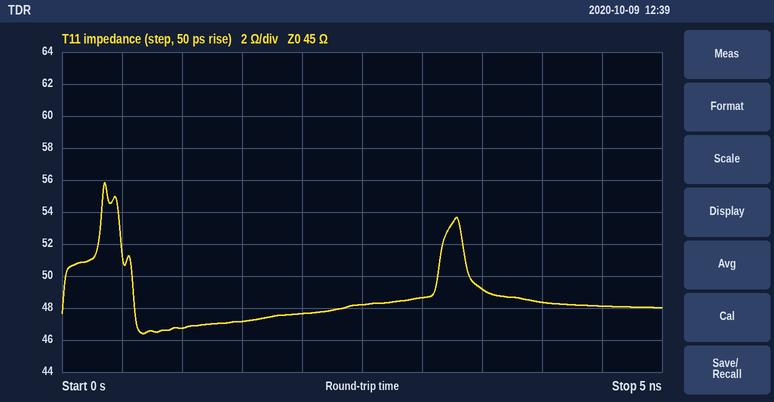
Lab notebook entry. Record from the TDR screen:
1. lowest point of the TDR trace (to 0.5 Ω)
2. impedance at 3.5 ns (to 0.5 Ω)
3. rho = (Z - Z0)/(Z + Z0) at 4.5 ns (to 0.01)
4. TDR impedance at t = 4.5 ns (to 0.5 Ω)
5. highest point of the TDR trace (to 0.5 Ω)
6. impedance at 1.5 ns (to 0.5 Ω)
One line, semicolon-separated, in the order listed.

46.5 Ω; 49.0 Ω; +0.03; 48.0 Ω; 56.0 Ω; 47.0 Ω
